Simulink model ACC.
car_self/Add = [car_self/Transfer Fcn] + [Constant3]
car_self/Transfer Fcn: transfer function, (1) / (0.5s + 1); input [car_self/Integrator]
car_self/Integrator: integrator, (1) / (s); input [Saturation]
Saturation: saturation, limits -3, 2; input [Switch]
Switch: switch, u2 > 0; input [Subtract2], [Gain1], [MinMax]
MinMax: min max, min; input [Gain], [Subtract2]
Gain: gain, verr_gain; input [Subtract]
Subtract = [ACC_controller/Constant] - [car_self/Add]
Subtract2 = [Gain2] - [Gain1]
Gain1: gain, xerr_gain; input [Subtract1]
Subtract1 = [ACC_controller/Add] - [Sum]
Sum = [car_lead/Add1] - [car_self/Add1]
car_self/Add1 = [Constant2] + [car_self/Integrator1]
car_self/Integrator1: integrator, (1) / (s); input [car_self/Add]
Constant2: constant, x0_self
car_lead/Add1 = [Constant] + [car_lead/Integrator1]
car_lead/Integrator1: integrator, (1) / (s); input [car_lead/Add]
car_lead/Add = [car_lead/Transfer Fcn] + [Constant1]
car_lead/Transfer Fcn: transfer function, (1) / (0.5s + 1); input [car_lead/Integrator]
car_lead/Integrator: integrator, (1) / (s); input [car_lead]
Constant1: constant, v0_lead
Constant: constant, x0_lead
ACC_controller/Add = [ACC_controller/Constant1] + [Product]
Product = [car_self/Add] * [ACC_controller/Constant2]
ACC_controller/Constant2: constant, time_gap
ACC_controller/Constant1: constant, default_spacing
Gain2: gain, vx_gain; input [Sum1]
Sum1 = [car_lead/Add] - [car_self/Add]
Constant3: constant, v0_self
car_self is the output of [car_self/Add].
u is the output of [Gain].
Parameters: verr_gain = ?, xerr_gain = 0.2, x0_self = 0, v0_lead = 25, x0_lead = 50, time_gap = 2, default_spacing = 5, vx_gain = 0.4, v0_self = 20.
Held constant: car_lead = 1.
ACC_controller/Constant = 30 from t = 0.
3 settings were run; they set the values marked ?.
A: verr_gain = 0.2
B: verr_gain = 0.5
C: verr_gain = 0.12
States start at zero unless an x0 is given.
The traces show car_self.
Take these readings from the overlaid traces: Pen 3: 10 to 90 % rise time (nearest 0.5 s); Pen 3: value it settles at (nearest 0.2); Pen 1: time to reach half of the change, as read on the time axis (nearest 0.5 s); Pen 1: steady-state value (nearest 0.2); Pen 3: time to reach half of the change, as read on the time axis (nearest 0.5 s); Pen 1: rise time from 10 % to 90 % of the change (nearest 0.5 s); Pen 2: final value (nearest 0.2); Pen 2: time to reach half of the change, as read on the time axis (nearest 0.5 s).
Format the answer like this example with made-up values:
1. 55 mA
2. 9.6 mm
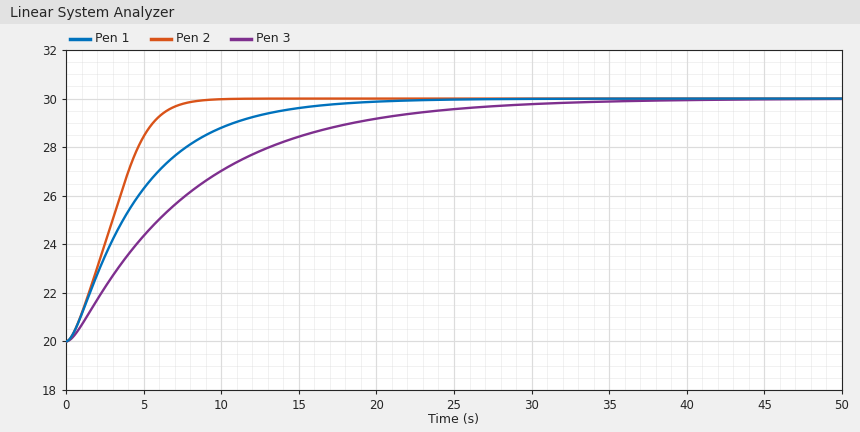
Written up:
1. 17.0 s
2. 30.0
3. 3.5 s
4. 30.0
5. 6.0 s
6. 10.0 s
7. 30.0
8. 3.0 s
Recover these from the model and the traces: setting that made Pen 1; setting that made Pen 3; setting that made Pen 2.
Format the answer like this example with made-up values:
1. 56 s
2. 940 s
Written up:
1. A
2. C
3. B
